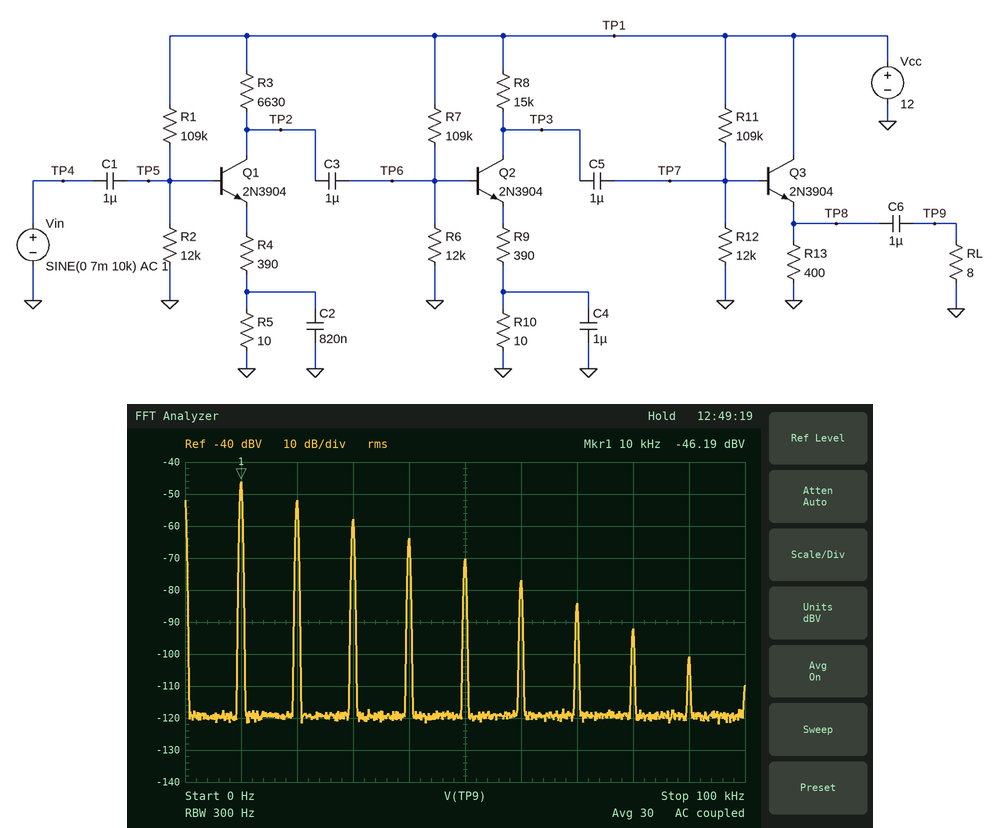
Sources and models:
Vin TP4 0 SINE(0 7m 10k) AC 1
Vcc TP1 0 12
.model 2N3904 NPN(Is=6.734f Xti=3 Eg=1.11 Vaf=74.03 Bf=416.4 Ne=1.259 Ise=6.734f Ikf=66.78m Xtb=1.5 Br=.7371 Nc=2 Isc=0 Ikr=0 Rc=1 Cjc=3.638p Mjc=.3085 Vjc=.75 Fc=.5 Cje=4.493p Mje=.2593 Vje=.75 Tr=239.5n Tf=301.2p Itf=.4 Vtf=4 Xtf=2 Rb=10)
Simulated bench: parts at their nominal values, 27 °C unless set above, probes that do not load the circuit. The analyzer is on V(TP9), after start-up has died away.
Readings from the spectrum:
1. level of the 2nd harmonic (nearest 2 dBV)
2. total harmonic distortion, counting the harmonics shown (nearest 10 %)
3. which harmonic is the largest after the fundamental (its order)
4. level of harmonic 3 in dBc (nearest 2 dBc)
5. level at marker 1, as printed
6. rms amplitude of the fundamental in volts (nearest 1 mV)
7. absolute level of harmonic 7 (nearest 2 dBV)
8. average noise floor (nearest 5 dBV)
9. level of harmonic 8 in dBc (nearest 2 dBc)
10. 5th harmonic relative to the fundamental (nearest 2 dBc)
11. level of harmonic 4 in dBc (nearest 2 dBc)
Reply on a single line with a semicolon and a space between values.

-52 dBV; 60 %; 2; -12 dBc; -46.19 dBV; 5 mV; -84 dBV; -120 dBV; -46 dBc; -24 dBc; -18 dBc
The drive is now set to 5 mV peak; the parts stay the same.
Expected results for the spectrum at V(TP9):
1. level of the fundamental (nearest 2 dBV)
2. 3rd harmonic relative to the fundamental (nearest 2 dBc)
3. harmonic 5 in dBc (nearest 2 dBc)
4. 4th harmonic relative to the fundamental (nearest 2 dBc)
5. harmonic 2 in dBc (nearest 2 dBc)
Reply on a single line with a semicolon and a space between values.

-52 dBV; -20 dBc; -40 dBc; -30 dBc; -10 dBc
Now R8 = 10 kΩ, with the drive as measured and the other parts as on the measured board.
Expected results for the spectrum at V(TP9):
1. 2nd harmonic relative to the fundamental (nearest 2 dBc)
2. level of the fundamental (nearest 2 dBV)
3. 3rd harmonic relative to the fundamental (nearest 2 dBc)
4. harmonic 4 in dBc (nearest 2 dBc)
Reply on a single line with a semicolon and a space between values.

-4 dBc; -34 dBV; -10 dBc; -24 dBc
